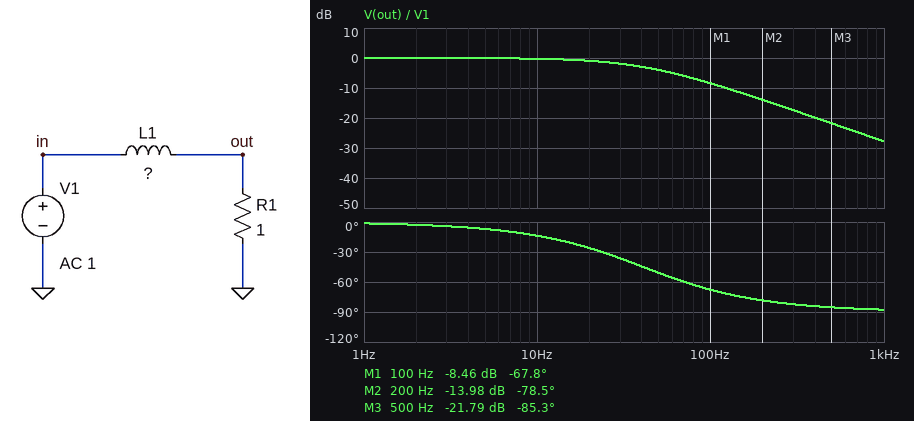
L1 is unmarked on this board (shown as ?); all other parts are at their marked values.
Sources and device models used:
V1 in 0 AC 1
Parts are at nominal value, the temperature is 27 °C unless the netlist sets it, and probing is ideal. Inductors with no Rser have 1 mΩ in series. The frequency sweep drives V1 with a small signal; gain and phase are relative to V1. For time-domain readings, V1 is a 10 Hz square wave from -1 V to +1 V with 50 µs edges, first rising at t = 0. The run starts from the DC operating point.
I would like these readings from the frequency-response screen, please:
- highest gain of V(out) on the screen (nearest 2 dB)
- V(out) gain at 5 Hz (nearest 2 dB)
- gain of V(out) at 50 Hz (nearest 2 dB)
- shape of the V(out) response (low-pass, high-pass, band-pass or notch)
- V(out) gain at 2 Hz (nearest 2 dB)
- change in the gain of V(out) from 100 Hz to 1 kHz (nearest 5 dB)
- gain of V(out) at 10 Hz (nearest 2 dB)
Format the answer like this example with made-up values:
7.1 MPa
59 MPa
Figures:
0 dB
0 dB
-4 dB
low-pass
0 dB
-20 dB
0 dB
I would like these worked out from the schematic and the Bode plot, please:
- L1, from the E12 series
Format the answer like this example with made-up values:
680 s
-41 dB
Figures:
3.9 mH
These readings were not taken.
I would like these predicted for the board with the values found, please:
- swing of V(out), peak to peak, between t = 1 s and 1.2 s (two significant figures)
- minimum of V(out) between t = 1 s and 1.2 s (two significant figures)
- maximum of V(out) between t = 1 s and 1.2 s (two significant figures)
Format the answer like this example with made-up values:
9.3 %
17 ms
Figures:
2.0 V
-1.0 V
1.0 V
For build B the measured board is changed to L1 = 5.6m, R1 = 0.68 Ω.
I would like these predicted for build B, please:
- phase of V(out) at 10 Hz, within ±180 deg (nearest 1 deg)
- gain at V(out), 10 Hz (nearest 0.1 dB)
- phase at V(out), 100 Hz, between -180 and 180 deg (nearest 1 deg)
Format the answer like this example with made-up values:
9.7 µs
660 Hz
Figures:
-27 deg
-1.0 dB
-79 deg
